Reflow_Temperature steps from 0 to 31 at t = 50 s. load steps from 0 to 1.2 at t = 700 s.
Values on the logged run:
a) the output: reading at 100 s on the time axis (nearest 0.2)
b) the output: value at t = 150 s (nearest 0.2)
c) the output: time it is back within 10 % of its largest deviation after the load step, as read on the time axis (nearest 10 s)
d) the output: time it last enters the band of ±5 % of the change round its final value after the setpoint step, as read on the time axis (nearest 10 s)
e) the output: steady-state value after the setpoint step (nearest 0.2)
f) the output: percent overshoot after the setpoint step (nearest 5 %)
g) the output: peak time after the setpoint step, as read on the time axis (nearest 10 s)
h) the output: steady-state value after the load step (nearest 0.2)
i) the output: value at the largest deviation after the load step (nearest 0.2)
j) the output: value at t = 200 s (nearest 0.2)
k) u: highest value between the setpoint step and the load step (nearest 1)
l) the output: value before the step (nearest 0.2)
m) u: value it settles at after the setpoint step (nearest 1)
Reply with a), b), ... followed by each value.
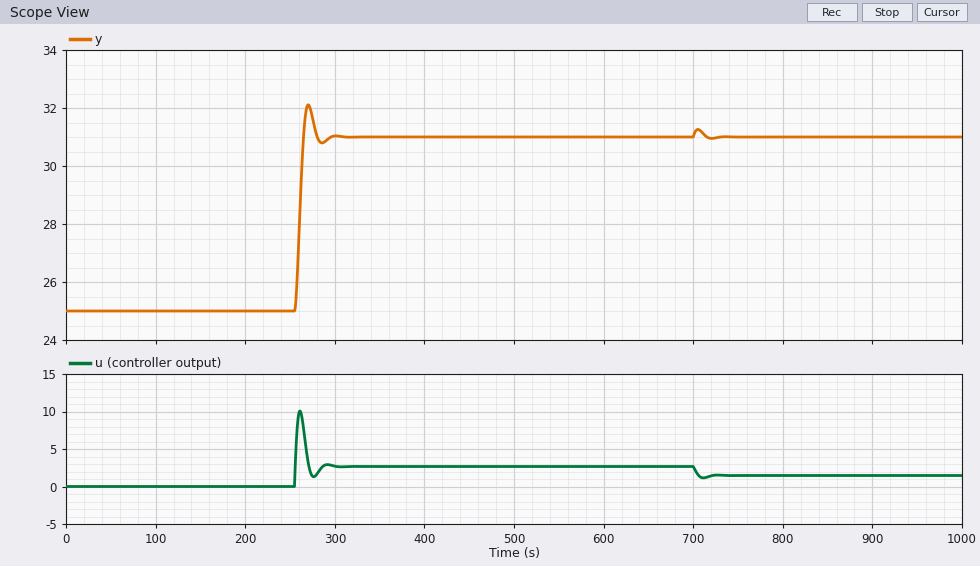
a) 25.0
b) 25.0
c) 730 s
d) 280 s
e) 31.0
f) 20 %
g) 270 s
h) 31.0
i) 31.2
j) 25.0
k) 10
l) 25.0
m) 3
